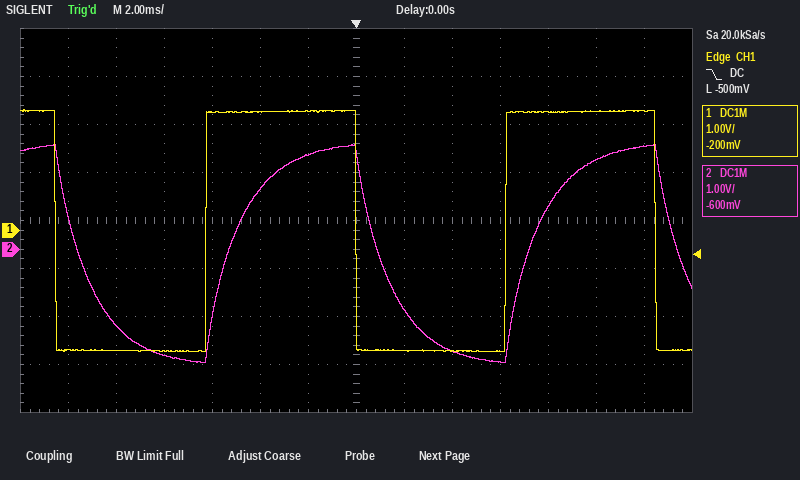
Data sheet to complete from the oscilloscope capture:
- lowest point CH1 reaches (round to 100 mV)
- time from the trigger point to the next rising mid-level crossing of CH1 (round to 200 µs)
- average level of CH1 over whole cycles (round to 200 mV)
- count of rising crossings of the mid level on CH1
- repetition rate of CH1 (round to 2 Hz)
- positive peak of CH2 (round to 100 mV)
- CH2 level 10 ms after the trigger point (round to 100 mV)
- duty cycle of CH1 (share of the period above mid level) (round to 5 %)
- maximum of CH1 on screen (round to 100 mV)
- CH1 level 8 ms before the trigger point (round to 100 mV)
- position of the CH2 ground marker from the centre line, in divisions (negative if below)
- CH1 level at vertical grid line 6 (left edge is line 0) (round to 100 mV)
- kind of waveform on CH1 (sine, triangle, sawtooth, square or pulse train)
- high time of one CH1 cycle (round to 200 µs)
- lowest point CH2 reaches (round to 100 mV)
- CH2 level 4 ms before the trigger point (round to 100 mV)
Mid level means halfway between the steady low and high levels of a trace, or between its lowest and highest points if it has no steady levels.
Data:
-2.5 V
6.2 ms
0.0 V
2
80 Hz
2.2 V
1.9 V
50 %
2.5 V
-2.5 V
-0.6 div
2.5 V
square
6.2 ms
-2.4 V
1.3 V
